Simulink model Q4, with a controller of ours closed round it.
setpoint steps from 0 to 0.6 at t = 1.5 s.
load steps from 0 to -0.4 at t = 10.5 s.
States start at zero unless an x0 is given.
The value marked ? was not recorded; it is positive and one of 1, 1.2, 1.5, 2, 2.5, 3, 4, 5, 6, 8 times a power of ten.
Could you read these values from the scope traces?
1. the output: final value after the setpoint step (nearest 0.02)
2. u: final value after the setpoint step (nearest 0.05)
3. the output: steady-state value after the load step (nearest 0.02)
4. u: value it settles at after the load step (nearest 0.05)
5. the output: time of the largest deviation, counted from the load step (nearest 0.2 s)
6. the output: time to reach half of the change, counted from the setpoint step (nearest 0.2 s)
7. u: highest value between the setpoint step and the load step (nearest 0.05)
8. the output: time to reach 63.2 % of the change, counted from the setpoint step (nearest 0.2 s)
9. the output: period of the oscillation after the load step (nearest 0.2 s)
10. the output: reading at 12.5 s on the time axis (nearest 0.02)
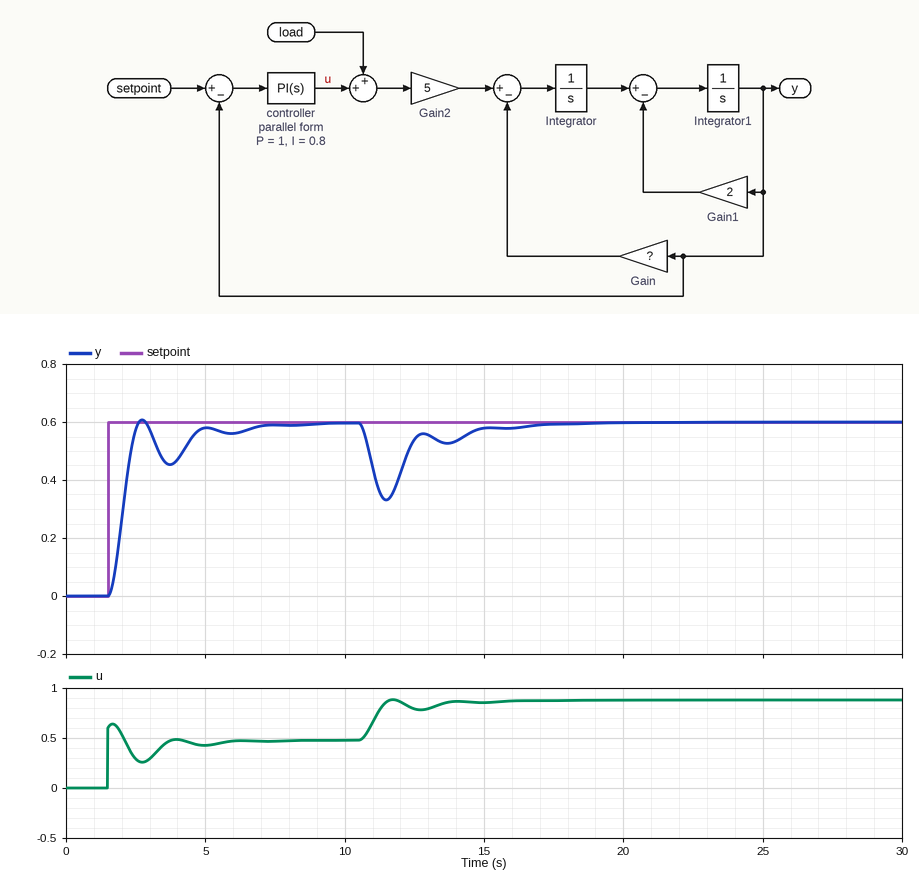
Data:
0.60
0.50
0.60
0.90
1.0 s
0.6 s
0.65
0.6 s
2.2 s
0.54
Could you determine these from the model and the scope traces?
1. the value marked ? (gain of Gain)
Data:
4
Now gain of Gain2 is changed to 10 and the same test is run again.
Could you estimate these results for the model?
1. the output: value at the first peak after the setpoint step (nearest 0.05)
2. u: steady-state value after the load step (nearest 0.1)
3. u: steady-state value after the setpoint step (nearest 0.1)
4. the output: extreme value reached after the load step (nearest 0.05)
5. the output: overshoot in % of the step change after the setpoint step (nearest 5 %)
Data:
0.75
0.6
0.2
0.25
25 %
